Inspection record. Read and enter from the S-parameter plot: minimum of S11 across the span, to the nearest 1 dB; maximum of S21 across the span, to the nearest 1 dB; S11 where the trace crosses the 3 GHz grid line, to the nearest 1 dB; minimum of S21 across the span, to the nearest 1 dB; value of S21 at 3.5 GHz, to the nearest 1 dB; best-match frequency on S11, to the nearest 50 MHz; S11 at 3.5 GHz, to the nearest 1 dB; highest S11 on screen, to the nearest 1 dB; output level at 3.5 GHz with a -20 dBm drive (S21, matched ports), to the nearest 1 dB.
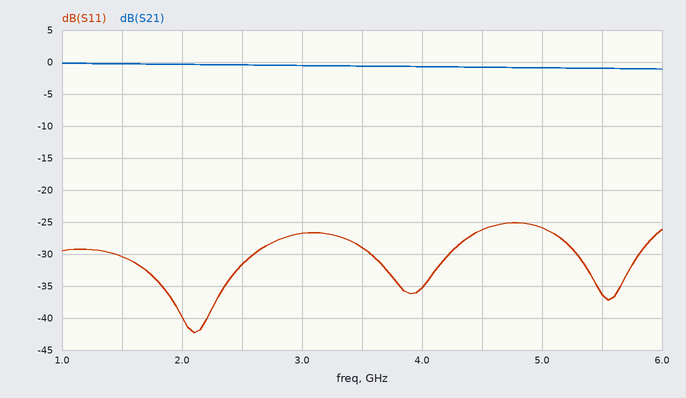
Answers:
-42 dB
0 dB
-27 dB
-1 dB
-1 dB
2.10 GHz
-29 dB
-25 dB
-21 dBm
